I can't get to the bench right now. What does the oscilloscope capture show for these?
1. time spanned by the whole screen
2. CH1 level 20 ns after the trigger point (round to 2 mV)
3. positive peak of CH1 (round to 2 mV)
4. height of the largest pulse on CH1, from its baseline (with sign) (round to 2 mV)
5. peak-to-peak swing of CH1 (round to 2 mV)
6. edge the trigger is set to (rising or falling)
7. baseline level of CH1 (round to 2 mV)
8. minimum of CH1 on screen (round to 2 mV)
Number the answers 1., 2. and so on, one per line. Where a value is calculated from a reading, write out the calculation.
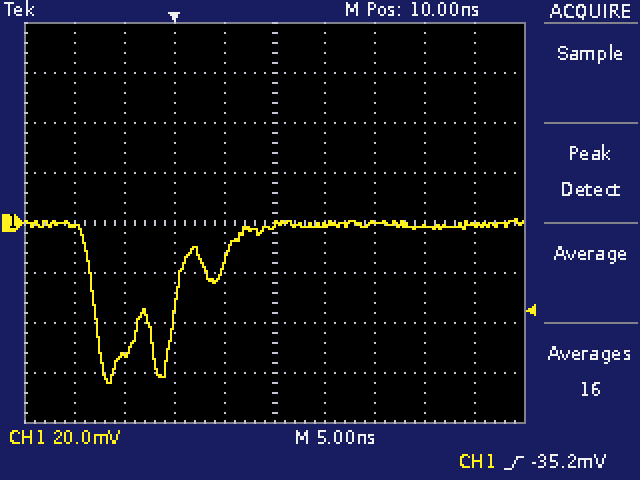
1. 50 ns
2. 0 mV
3. 2 mV
4. -64 mV − (0 mV) = -64 mV
5. 2 mV − (-64 mV) = 66 mV
6. rising
7. 0 mV
8. -64 mV
